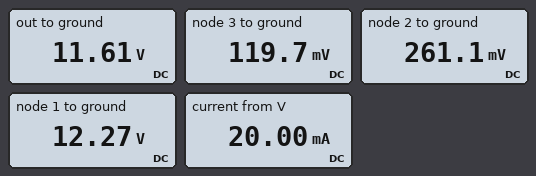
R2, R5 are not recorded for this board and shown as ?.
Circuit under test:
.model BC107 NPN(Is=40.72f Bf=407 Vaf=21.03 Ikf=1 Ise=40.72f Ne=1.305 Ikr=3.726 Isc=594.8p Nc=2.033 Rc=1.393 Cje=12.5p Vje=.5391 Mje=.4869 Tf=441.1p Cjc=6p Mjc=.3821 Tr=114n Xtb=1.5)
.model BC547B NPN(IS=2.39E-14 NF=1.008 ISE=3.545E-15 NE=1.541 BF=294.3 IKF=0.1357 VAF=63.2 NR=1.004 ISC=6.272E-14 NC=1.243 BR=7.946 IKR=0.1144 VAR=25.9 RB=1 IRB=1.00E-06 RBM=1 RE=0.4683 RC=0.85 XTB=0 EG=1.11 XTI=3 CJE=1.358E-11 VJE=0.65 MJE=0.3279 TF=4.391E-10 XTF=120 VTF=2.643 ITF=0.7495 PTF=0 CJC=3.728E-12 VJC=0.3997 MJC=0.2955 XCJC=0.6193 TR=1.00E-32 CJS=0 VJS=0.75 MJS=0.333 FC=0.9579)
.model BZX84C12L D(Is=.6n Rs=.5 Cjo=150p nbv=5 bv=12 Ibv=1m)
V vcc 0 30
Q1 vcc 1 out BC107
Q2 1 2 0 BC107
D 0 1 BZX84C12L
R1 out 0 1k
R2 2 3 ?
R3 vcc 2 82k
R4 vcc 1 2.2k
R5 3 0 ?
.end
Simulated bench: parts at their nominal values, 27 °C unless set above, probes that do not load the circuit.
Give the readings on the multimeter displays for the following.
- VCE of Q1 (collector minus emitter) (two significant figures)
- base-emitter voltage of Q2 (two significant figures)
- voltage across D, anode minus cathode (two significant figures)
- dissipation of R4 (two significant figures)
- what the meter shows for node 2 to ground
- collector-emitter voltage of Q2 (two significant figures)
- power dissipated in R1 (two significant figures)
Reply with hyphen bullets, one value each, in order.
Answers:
- 18 V
- 260 mV
- -12 V
- 140 mW
- 261.1 mV
- 12 V
- 130 mW
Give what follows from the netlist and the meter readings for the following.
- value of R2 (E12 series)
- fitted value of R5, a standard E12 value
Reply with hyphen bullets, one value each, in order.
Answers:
- 390 Ω
- 330 Ω
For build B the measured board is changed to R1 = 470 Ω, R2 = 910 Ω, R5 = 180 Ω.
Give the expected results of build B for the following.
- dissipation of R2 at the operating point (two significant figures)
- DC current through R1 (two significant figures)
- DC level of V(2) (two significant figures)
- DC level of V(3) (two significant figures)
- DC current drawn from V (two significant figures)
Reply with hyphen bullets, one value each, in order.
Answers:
- 120 µW
- 25 mA
- 390 mV
- 65 mV
- 33 mA
